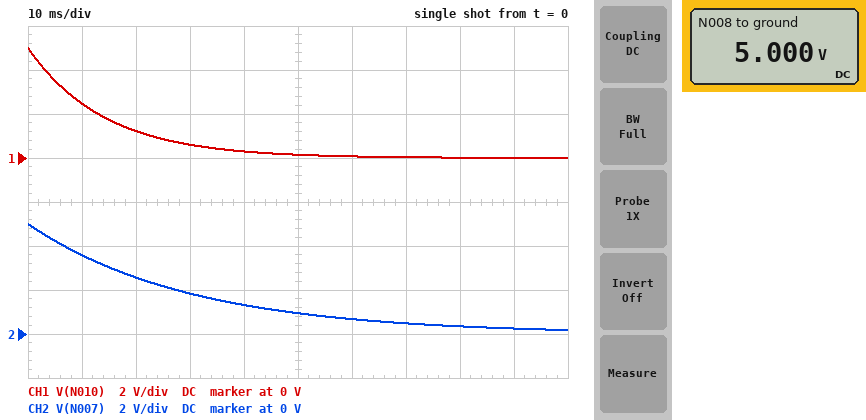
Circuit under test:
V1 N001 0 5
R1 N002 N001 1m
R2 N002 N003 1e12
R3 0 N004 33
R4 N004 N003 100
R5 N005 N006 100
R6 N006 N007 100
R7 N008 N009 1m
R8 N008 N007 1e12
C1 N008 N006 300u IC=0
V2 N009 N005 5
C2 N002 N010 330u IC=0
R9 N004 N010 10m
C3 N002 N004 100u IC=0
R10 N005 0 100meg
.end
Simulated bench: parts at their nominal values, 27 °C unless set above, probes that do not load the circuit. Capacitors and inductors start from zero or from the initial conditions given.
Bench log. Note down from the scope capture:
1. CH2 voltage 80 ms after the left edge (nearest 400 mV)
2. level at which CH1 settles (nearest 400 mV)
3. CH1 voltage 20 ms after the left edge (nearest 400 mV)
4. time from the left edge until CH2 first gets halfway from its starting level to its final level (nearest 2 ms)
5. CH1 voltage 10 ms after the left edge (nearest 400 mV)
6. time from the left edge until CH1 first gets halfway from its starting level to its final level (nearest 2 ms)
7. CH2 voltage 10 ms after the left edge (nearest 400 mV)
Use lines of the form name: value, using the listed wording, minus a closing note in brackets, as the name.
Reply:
CH2 voltage 80 ms after the left edge: 400 mV
level at which CH1 settles: 0 V
CH1 voltage 20 ms after the left edge: 1.2 V
time from the left edge until CH2 first gets halfway from its starting level to its final level: 20 ms
CH1 voltage 10 ms after the left edge: 2.4 V
time from the left edge until CH1 first gets halfway from its starting level to its final level: 10 ms
CH2 voltage 10 ms after the left edge: 3.6 V
